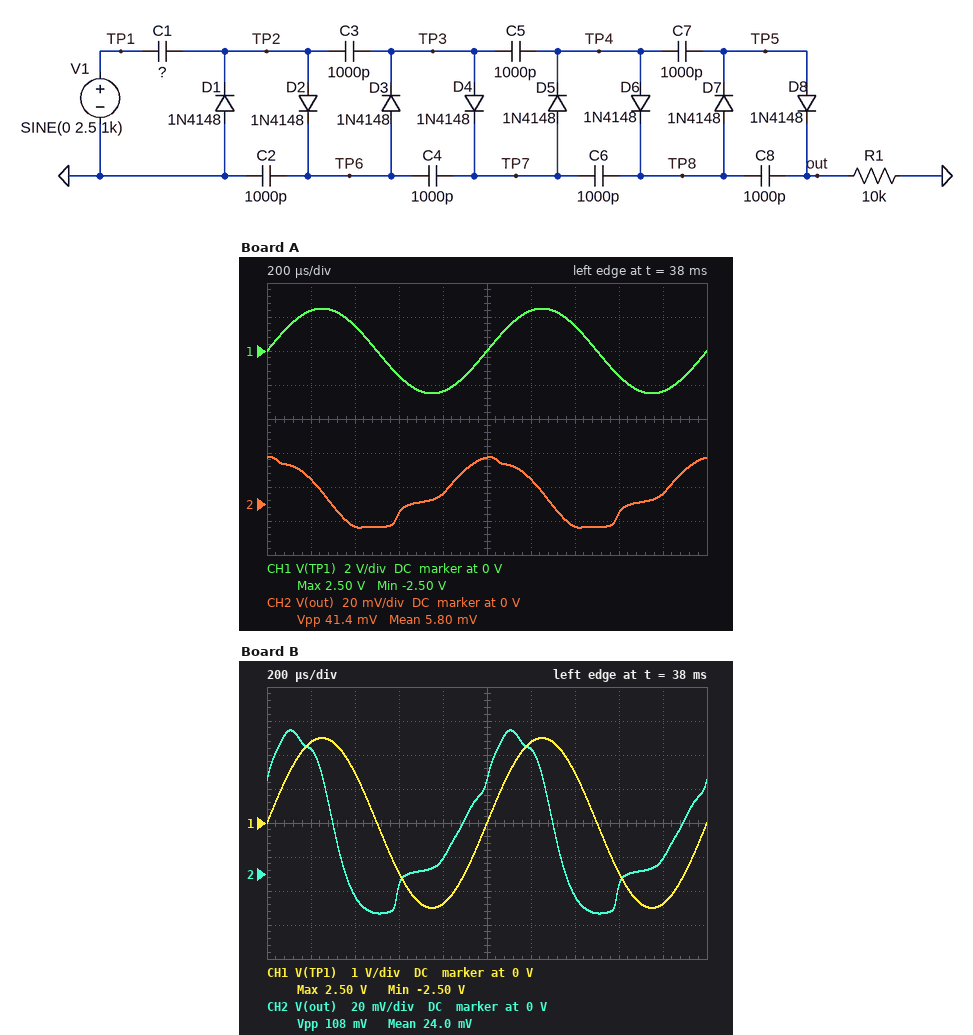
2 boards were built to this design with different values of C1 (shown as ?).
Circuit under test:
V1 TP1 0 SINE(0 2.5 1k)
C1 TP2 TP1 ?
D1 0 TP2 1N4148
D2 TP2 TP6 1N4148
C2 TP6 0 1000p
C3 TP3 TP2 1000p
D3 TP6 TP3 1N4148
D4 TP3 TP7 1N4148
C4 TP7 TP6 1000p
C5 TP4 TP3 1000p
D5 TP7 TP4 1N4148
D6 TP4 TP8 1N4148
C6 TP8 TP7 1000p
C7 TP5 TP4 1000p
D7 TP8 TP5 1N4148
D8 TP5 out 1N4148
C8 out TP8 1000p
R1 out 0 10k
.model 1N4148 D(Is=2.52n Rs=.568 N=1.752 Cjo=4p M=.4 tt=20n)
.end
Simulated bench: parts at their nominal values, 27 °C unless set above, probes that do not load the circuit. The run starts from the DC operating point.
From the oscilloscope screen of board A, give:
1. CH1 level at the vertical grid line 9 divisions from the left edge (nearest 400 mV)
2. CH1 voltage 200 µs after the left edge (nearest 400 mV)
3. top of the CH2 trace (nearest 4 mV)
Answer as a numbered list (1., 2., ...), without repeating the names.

1. -2.4 V
2. 2.4 V
3. 28 mV
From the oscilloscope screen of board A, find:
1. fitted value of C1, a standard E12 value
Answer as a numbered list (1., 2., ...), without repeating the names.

1. 470 pF
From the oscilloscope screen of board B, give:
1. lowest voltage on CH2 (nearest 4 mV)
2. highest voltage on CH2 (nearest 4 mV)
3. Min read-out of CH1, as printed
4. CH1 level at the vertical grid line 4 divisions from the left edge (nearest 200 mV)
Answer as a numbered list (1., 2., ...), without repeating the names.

1. -24 mV
2. 84 mV
3. -2.50 V
4. -2.4 V
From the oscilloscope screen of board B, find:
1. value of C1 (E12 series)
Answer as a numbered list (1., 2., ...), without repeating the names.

1. 1.8 nF
